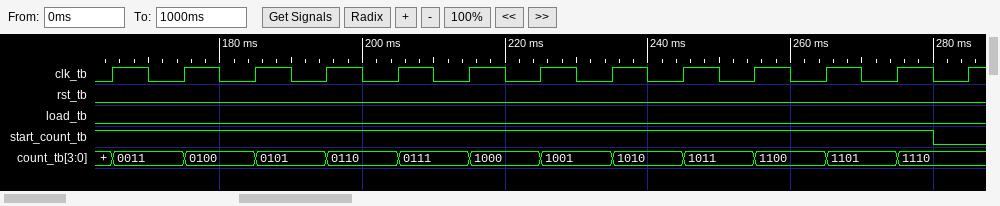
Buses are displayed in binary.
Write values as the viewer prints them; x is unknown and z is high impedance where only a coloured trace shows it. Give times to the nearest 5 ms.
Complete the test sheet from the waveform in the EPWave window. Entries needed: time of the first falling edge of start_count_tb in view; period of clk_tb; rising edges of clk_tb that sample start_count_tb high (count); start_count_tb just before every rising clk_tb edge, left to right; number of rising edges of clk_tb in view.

280 ms
10 ms
12
1 1 1 1 1 1 1 1 1 1 1 1 0
13
